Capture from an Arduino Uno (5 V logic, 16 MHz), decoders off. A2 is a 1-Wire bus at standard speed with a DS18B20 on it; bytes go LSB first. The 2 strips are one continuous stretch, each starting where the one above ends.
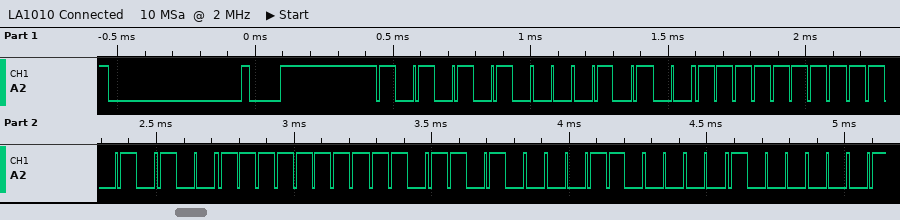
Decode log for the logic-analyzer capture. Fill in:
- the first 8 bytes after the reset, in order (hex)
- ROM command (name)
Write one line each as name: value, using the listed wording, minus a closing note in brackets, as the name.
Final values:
the first 8 bytes after the reset, in order: 55 28 FF 2B FF 5B 18 04
ROM command: Match ROM
